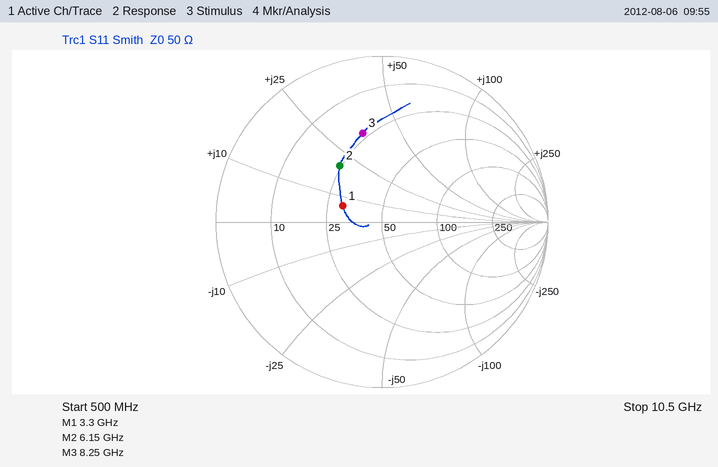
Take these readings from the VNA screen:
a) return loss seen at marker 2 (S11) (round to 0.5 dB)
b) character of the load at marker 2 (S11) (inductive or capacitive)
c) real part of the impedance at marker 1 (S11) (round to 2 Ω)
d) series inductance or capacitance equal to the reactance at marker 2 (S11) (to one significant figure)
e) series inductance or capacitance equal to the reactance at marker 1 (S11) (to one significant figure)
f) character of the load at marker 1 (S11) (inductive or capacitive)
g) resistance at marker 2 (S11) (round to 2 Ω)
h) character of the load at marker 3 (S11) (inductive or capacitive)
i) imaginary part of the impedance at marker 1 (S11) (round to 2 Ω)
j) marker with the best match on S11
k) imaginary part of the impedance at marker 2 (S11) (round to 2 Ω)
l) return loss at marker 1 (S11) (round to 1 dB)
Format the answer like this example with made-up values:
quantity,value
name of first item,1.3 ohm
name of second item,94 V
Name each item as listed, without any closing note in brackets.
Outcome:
quantity,value
return loss seen at marker 2 (S11),7.5 dB
character of the load at marker 2 (S11),inductive
real part of the impedance at marker 1 (S11),30 Ω
series inductance or capacitance equal to the reactance at marker 2 (S11),500 pH
series inductance or capacitance equal to the reactance at marker 1 (S11),300 pH
character of the load at marker 1 (S11),inductive
resistance at marker 2 (S11),24 Ω
character of the load at marker 3 (S11),inductive
imaginary part of the impedance at marker 1 (S11),+6 Ω
marker with the best match on S11,marker 1
imaginary part of the impedance at marker 2 (S11),+20 Ω
return loss at marker 1 (S11),12 dB
